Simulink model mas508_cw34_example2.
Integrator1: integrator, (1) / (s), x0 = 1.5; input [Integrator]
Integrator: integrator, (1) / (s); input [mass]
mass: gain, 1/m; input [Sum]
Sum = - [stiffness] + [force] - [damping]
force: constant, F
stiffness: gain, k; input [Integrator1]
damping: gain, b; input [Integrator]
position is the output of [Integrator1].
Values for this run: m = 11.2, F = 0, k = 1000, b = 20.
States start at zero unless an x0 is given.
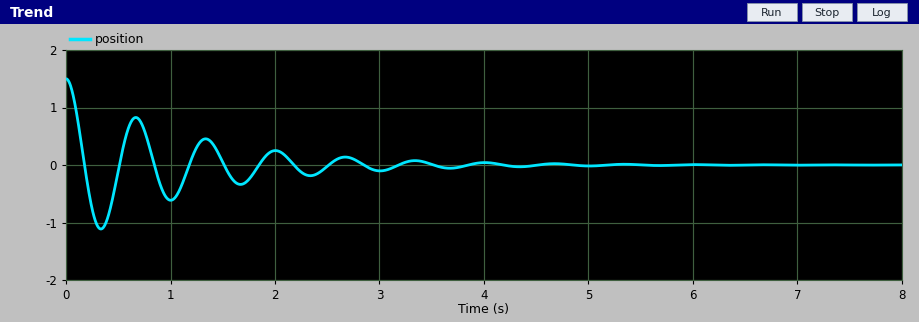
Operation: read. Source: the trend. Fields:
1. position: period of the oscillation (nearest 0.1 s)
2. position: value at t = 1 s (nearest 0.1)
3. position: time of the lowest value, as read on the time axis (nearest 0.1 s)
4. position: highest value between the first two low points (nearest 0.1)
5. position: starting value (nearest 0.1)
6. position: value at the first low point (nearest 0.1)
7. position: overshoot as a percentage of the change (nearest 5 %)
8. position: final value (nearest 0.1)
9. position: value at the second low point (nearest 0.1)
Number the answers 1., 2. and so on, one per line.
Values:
1. 0.7 s
2. -0.6
3. 0.3 s
4. 0.8
5. 1.5
6. -1.1
7. 75 %
8. 0.0
9. -0.6
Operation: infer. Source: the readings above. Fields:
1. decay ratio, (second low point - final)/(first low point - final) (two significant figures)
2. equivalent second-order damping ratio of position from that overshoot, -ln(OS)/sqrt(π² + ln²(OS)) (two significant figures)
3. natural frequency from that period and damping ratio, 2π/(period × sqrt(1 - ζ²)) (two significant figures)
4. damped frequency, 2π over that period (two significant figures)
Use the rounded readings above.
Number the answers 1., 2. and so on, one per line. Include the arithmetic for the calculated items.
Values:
1. (-0.6 - 0) / (-1.1 - 0) = 0.55
2. ln(0.75) = -0.288; 0.288 / sqrt(9.870 + 0.083) = 0.091
3. 2π / (0.7 × sqrt(1 - 0.091²)) = 9.0 rad/s
4. 2π / 0.7 = 9.0 rad/s
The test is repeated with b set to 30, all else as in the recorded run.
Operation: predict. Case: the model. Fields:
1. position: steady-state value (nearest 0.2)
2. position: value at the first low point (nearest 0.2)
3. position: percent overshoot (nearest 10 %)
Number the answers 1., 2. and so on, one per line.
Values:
1. 0.0
2. -1.0
3. 60 %
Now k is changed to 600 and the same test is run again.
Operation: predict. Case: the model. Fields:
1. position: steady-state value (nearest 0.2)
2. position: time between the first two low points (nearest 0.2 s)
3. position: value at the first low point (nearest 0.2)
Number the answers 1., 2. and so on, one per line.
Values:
1. 0.0
2. 0.8 s
3. -1.0
